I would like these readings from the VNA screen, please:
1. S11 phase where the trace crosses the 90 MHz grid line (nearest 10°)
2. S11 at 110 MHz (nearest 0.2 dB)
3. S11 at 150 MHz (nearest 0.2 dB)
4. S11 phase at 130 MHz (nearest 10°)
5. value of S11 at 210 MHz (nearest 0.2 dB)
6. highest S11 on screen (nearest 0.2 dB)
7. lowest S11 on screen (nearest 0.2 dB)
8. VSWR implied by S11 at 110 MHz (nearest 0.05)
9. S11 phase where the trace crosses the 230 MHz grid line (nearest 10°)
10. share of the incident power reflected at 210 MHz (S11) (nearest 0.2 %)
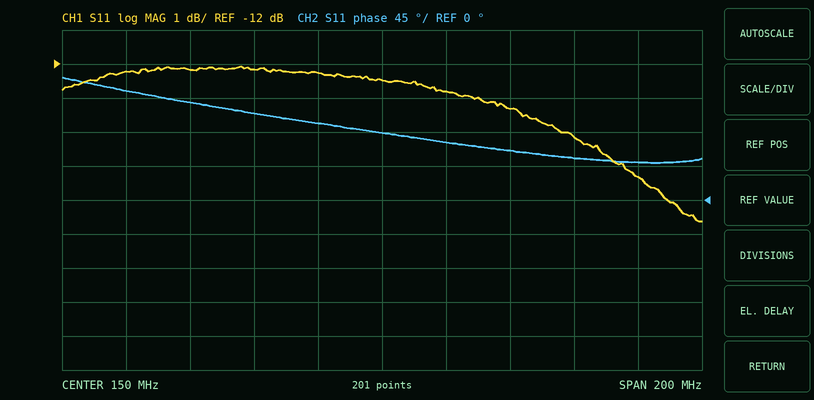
130°
-12.2 dB
-12.4 dB
100°
-14.2 dB
-12.0 dB
-16.6 dB
1.65
50°
3.8 %
